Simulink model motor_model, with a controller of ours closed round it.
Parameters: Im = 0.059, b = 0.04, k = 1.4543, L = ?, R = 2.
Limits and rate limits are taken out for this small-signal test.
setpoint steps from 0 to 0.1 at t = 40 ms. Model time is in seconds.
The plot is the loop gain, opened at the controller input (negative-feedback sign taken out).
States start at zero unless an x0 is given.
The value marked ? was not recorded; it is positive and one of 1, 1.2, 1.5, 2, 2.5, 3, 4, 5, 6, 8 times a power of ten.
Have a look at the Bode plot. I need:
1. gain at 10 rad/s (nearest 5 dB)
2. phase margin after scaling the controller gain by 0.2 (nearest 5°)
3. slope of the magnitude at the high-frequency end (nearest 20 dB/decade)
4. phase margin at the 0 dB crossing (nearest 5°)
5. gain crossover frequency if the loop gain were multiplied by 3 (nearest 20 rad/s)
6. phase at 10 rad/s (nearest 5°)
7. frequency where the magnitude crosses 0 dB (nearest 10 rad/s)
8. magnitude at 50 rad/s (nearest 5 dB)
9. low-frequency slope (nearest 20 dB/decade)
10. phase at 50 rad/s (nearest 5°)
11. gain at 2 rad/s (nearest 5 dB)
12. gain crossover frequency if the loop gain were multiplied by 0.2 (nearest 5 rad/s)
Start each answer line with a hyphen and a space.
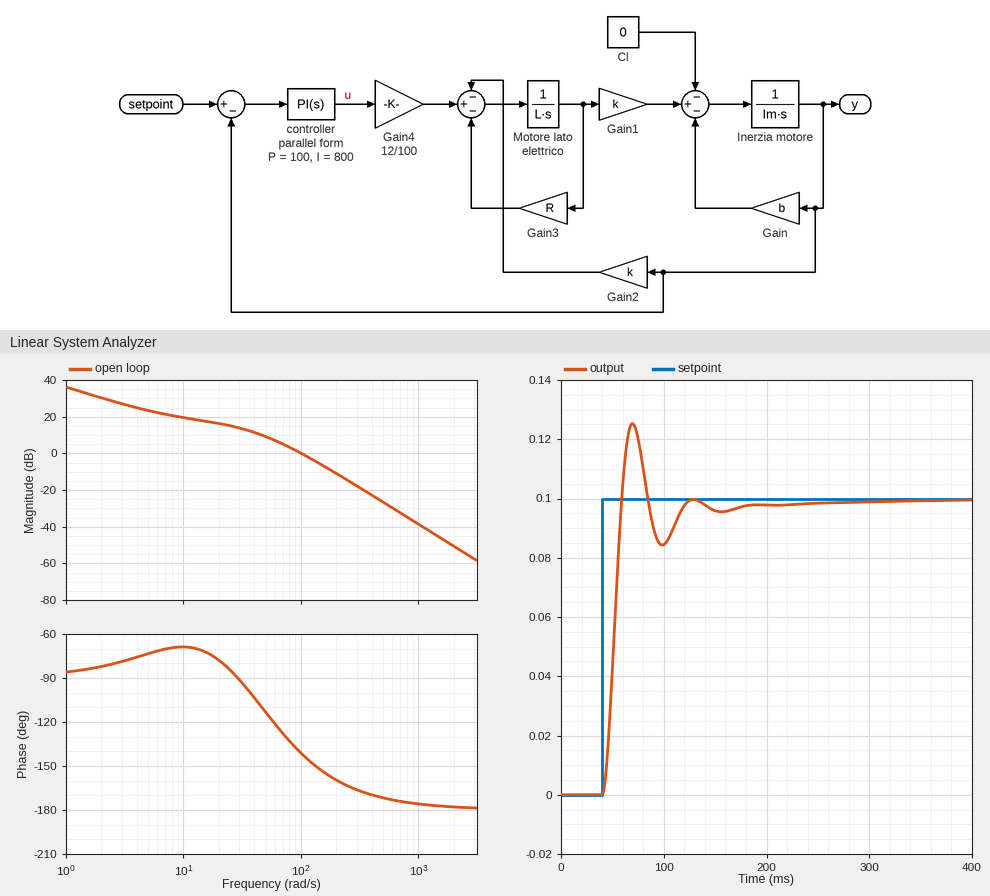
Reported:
- 20 dB
- 90°
- -40 dB/decade
- 40°
- 180 rad/s
- -70°
- 100 rad/s
- 10 dB
- -20 dB/decade
- -115°
- 30 dB
- 30 rad/s
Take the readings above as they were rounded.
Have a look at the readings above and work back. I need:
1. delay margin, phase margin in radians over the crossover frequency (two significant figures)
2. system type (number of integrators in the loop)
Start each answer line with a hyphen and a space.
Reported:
- 0.0070 s
- 1
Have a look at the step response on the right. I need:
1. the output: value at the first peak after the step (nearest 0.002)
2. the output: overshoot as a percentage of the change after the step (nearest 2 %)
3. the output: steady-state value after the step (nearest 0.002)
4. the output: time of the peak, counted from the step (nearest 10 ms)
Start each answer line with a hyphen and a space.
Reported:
- 0.126
- 26 %
- 0.100
- 30 ms
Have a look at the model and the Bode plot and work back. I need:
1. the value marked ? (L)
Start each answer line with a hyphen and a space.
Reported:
- 0.025
